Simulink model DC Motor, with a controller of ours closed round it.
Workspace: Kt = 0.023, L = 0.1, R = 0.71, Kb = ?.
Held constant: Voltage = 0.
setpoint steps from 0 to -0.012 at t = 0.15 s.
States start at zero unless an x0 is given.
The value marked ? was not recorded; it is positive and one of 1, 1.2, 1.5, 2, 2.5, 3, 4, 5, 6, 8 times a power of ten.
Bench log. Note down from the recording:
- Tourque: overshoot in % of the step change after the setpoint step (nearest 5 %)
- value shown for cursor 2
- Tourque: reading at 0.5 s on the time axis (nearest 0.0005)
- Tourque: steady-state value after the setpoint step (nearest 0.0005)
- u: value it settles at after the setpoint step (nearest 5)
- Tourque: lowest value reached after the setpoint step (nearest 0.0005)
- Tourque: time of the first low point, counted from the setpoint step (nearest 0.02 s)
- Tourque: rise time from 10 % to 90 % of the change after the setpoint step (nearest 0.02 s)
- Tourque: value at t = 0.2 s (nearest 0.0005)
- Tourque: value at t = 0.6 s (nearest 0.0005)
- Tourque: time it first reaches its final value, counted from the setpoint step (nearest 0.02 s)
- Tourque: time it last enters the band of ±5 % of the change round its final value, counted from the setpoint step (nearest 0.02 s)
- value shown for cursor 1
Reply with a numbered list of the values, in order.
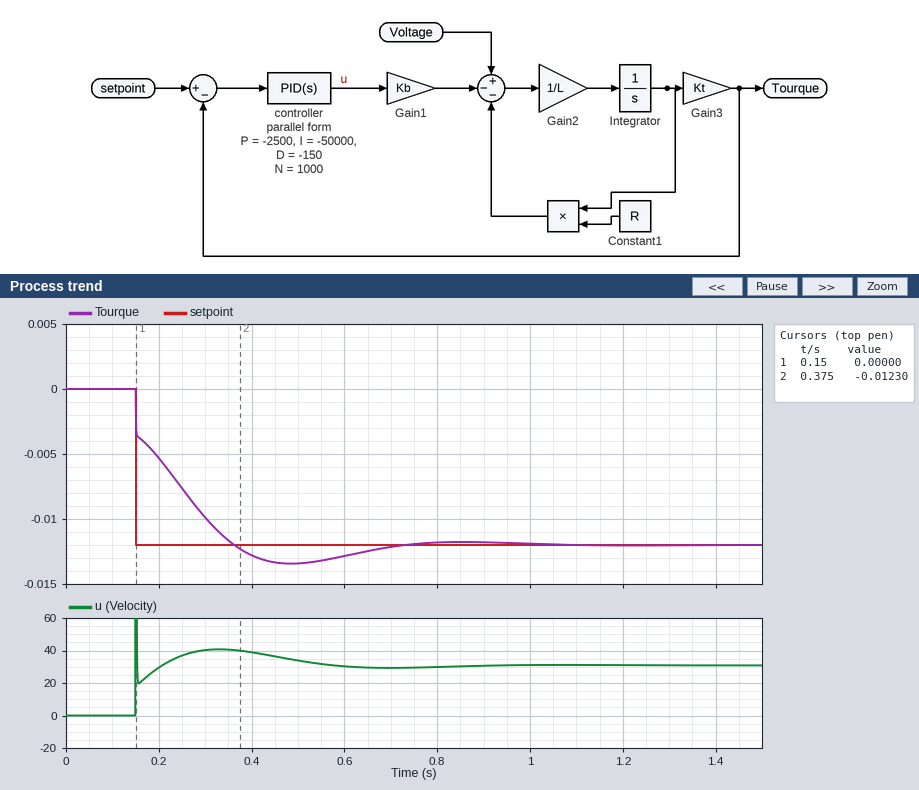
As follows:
1. 10 %
2. -0.01230
3. -0.0135
4. -0.0120
5. 30
6. -0.0135
7. 0.34 s
8. 0.18 s
9. -0.0055
10. -0.0130
11. 0.22 s
12. 0.48 s
13. 0.00000
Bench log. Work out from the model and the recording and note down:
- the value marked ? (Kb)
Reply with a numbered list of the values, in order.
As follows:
1. 0.012
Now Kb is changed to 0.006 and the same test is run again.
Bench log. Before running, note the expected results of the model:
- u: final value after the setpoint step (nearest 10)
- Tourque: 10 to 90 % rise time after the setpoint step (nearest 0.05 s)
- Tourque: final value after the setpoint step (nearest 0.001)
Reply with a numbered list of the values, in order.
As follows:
1. 60
2. 0.25 s
3. -0.012
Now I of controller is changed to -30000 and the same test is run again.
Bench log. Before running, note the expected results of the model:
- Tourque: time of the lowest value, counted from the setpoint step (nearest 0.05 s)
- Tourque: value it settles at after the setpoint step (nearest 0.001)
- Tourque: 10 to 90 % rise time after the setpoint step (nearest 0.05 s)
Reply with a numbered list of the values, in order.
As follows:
1. 0.50 s
2. -0.012
3. 0.25 s
